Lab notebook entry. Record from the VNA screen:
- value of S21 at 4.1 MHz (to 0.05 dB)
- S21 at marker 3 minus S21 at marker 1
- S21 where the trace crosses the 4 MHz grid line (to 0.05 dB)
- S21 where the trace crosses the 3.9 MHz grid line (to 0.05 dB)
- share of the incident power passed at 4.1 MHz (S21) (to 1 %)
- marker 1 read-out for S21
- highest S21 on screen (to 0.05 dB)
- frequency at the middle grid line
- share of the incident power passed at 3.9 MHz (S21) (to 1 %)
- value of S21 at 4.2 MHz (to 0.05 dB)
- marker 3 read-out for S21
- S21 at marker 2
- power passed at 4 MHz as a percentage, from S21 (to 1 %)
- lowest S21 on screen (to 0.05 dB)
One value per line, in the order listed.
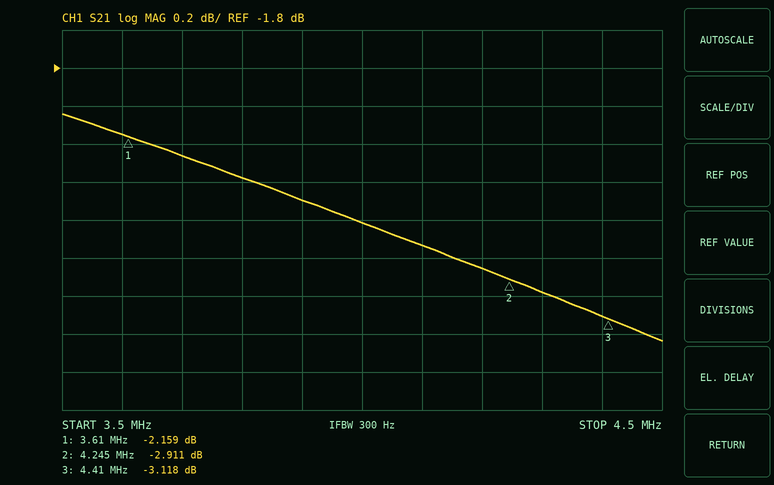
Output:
-2.75 dB
-0.959 dB
-2.60 dB
-2.50 dB
53 %
-2.159 dB
-2.05 dB
4 MHz
56 %
-2.85 dB
-3.118 dB
-2.911 dB
55 %
-3.25 dB
